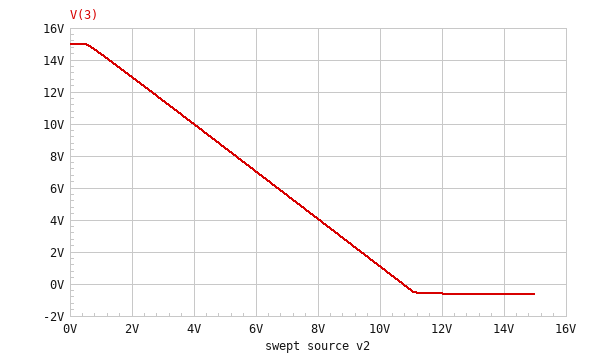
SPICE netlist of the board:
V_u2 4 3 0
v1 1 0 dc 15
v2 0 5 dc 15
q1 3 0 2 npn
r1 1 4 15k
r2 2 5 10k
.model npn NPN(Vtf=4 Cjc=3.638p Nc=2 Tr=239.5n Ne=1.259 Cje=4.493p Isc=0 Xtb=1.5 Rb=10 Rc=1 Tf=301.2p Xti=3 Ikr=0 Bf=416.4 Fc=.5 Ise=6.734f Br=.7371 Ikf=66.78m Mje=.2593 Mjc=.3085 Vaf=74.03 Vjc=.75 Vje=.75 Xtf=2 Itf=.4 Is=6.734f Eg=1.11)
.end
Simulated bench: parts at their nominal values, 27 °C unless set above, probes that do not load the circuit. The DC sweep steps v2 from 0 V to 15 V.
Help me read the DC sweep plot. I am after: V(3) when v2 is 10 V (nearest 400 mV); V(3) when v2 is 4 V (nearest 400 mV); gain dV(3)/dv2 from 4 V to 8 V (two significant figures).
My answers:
1.2 V
10.0 V
-1.5 V/V
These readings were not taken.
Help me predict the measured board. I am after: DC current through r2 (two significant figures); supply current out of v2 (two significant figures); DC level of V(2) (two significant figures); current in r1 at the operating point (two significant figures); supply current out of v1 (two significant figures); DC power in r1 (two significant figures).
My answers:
1.4 mA
1.4 mA
-680 mV
1.0 mA
1.0 mA
16 mW
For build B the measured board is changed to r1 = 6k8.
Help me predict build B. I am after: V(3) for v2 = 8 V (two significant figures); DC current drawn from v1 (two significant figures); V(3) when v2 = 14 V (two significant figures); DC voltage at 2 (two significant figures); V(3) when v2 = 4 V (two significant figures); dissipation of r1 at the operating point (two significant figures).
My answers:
10 V
1.4 mA
6.0 V
-670 mV
13 V
14 mW
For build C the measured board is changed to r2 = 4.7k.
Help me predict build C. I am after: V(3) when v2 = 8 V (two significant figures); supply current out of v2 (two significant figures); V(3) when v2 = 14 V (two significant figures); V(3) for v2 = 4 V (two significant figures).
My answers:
-640 mV
3.0 mA
-690 mV
4.4 V
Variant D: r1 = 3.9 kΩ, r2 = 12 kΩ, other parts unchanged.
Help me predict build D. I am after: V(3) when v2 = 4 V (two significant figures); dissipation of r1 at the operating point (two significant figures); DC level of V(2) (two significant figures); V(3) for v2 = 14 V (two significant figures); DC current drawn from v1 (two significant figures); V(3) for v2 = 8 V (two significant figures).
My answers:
14 V
5.5 mW
-670 mV
11 V
1.2 mA
13 V
